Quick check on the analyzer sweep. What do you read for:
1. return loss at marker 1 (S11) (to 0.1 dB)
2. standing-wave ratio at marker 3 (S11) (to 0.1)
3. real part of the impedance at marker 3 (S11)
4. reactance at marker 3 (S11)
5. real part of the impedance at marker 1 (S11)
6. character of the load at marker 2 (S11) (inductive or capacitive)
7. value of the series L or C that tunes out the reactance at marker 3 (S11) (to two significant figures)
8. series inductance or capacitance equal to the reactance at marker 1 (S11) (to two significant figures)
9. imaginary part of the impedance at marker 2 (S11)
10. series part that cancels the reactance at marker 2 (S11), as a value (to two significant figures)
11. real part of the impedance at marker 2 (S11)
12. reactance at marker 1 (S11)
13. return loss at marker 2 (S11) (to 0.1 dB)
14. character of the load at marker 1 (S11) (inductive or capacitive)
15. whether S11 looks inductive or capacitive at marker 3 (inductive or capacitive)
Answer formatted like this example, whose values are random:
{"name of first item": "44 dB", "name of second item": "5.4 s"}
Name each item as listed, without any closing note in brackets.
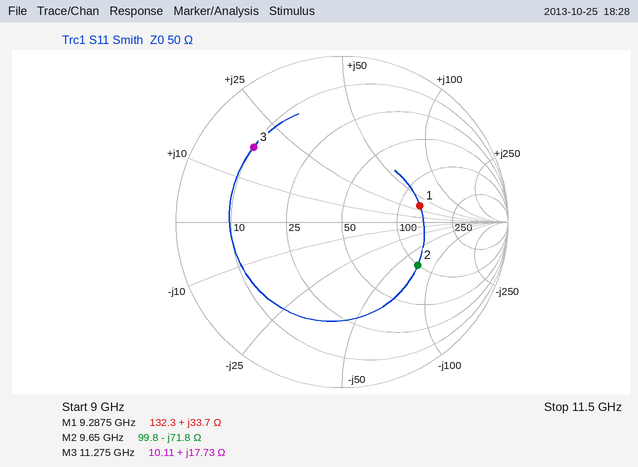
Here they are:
{"return loss at marker 1 (S11)": "6.4 dB", "standing-wave ratio at marker 3 (S11)": "5.6", "real part of the impedance at marker 3": "10.11 Ω", "reactance at marker 3": "+17.73 Ω", "real part of the impedance at marker 1": "132.3 Ω", "character of the load at marker 2 (S11)": "capacitive", "value of the series L or C that tunes out the reactance at marker 3 (S11)": "800 fF", "series inductance or capacitance equal to the reactance at marker 1 (S11)": "580 pH", "imaginary part of the impedance at marker 2": "-71.8 Ω", "series part that cancels the reactance at marker 2 (S11), as a value": "1.2 nH", "real part of the impedance at marker 2": "99.8 Ω", "reactance at marker 1": "+33.7 Ω", "return loss at marker 2 (S11)": "5.6 dB", "character of the load at marker 1 (S11)": "inductive", "whether S11 looks inductive or capacitive at marker 3": "inductive"}
